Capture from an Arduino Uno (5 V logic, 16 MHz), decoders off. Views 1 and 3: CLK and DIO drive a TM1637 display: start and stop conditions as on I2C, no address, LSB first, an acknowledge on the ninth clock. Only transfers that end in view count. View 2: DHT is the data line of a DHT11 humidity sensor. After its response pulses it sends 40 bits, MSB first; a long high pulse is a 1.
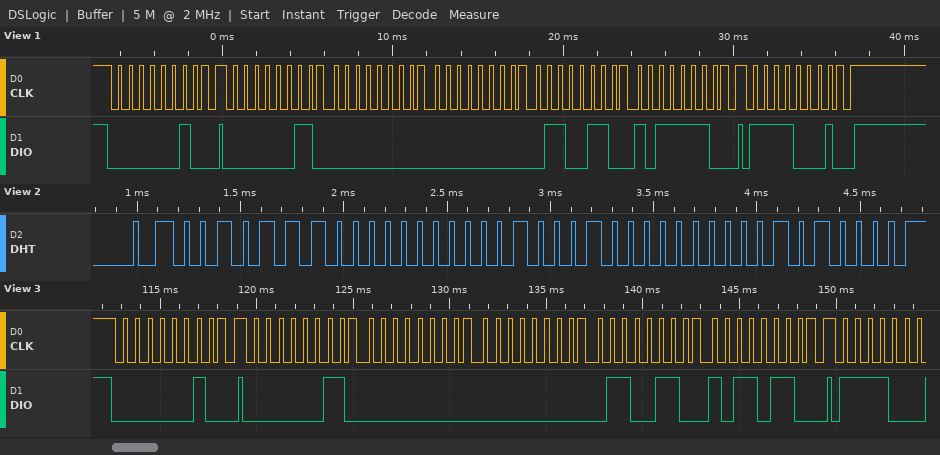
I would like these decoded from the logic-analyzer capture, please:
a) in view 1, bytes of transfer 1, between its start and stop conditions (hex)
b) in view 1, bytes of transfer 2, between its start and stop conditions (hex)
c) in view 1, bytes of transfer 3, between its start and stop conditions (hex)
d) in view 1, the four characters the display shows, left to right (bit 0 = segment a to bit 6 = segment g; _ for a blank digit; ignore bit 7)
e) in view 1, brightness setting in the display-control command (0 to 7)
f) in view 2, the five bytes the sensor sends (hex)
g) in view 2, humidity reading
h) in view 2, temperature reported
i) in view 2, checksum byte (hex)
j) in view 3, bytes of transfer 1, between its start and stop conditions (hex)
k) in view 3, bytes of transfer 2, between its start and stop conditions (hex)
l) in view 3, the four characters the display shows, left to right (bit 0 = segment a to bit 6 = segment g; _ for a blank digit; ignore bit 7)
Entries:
40
C0 00 00 66 7D
8F
__46
7
2E 00 22 00 50
46 %
34.0 °C
0x50
40
C0 00 00 66 6D
__45
